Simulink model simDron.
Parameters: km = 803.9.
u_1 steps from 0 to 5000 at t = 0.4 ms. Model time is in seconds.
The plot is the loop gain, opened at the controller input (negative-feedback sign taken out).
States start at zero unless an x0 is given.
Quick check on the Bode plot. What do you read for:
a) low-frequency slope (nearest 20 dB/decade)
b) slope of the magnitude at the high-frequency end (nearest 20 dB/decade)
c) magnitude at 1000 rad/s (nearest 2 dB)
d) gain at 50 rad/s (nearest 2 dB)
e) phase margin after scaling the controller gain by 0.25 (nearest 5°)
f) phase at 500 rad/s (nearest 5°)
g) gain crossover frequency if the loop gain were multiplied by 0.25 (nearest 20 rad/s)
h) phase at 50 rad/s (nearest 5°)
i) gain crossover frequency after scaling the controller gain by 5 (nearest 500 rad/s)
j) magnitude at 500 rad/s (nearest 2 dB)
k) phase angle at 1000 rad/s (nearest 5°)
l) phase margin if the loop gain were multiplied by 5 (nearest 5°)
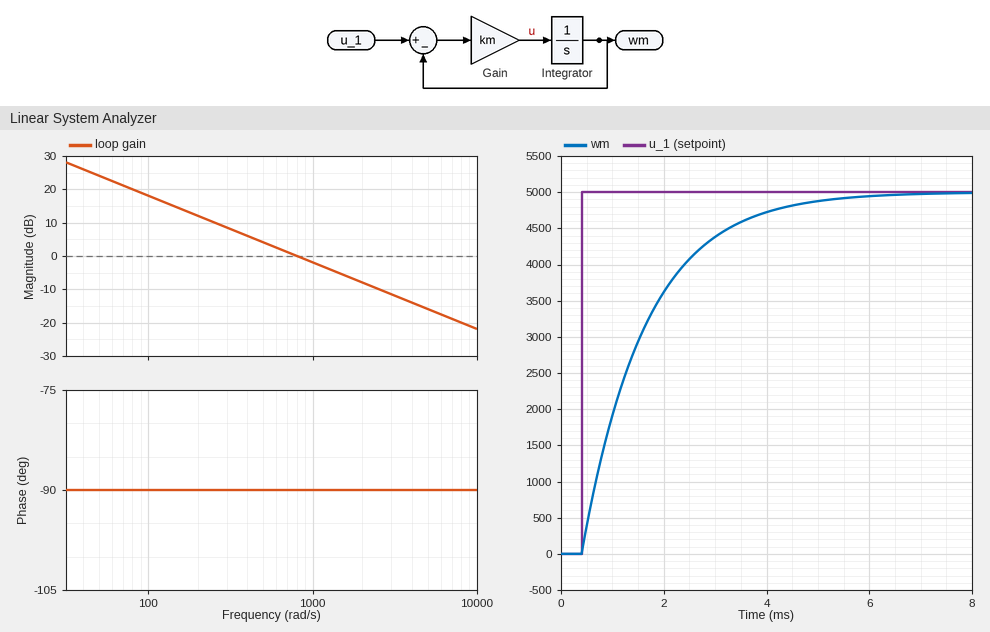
-20 dB/decade
-20 dB/decade
-2 dB
24 dB
90°
-90°
200 rad/s
-90°
4000 rad/s
4 dB
-90°
90°
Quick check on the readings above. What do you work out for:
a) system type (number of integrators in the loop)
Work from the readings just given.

1
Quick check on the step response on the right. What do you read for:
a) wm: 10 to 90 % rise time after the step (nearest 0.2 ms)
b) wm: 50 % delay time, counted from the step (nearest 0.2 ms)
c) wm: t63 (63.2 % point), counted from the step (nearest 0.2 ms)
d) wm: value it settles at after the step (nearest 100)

2.8 ms
0.8 ms
1.2 ms
5000
